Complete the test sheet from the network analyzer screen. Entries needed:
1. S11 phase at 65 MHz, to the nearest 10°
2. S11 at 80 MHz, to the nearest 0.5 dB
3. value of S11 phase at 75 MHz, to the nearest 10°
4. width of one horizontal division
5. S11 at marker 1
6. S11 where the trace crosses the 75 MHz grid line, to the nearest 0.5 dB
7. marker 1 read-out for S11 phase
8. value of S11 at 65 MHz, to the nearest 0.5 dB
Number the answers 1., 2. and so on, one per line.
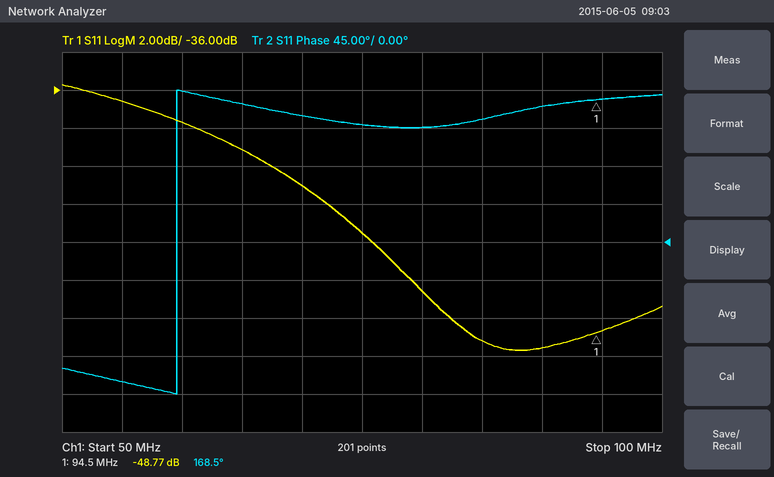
1. 160°
2. -46.5 dB
3. 140°
4. 5 MHz
5. -48.77 dB
6. -43.5 dB
7. 168.5°
8. -39.0 dB
